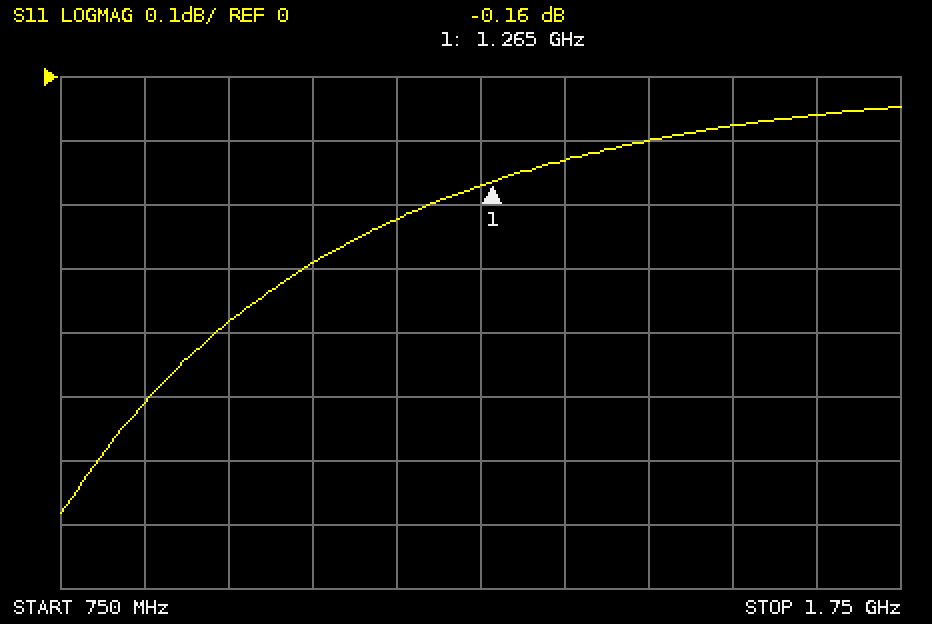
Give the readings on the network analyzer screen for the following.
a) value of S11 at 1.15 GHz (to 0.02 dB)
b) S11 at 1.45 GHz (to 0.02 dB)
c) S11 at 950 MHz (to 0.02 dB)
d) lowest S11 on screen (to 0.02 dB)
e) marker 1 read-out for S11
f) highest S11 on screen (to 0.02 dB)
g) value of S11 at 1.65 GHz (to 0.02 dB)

-0.22 dB
-0.10 dB
-0.38 dB
-0.68 dB
-0.16 dB
-0.04 dB
-0.06 dB
